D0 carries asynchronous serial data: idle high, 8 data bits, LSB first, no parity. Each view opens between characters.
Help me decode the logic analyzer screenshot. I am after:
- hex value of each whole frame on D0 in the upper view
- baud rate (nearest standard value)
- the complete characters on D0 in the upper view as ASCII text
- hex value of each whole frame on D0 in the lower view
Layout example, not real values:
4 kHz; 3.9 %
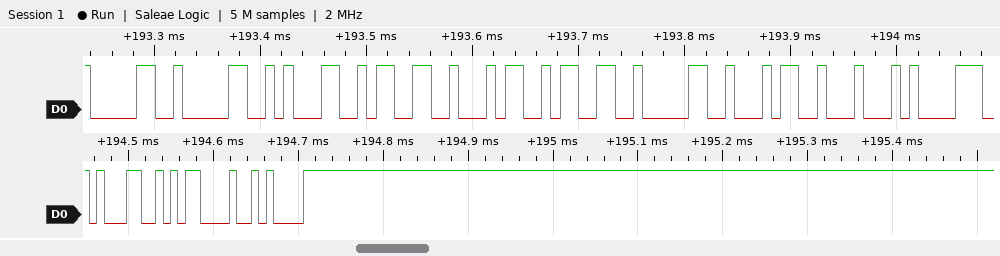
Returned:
30, 30, 31, 33, 34, 33, 30, 34, 44; 115200 baud; "00134304D"; 31, 0D, 0A
